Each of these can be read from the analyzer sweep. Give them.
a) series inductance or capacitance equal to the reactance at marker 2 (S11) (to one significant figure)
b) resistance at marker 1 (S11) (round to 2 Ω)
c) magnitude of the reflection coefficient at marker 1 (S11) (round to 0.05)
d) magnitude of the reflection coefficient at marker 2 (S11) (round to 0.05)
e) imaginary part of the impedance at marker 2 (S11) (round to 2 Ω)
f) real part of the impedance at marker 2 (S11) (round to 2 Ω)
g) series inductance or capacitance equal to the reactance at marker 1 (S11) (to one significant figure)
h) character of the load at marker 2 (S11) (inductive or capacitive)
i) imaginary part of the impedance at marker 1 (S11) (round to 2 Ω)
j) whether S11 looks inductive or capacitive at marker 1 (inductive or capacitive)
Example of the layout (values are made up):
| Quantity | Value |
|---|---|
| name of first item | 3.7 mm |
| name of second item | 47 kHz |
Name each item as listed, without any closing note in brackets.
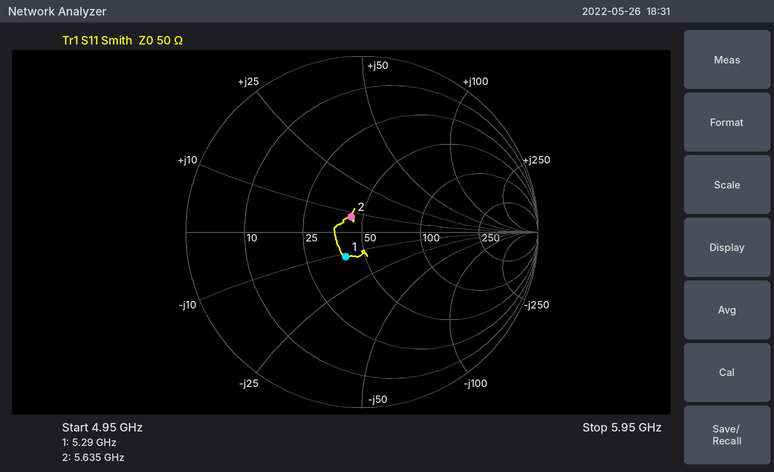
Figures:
| Quantity | Value |
|---|---|
| series inductance or capacitance equal to the reactance at marker 2 (S11) | 200 pH |
| resistance at marker 1 (S11) | 40 Ω |
| magnitude of the reflection coefficient at marker 1 (S11) | 0.15 |
| magnitude of the reflection coefficient at marker 2 (S11) | 0.10 |
| imaginary part of the impedance at marker 2 (S11) | +8 Ω |
| real part of the impedance at marker 2 (S11) | 44 Ω |
| series inductance or capacitance equal to the reactance at marker 1 (S11) | 3 pF |
| character of the load at marker 2 (S11) | inductive |
| imaginary part of the impedance at marker 1 (S11) | -12 Ω |
| whether S11 looks inductive or capacitive at marker 1 | capacitive |
